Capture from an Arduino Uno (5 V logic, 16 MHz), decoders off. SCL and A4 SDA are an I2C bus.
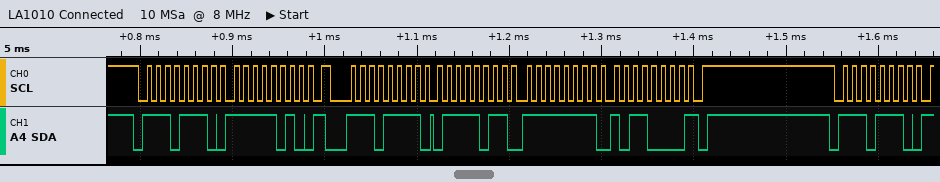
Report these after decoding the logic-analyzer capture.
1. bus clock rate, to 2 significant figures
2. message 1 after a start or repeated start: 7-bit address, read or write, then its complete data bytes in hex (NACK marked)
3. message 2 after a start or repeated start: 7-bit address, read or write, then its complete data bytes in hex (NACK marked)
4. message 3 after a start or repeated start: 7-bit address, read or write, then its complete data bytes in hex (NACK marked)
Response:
100 kHz
0x77 write: FA
0x77 read: 7B FF B0 NACK
0x77 write
